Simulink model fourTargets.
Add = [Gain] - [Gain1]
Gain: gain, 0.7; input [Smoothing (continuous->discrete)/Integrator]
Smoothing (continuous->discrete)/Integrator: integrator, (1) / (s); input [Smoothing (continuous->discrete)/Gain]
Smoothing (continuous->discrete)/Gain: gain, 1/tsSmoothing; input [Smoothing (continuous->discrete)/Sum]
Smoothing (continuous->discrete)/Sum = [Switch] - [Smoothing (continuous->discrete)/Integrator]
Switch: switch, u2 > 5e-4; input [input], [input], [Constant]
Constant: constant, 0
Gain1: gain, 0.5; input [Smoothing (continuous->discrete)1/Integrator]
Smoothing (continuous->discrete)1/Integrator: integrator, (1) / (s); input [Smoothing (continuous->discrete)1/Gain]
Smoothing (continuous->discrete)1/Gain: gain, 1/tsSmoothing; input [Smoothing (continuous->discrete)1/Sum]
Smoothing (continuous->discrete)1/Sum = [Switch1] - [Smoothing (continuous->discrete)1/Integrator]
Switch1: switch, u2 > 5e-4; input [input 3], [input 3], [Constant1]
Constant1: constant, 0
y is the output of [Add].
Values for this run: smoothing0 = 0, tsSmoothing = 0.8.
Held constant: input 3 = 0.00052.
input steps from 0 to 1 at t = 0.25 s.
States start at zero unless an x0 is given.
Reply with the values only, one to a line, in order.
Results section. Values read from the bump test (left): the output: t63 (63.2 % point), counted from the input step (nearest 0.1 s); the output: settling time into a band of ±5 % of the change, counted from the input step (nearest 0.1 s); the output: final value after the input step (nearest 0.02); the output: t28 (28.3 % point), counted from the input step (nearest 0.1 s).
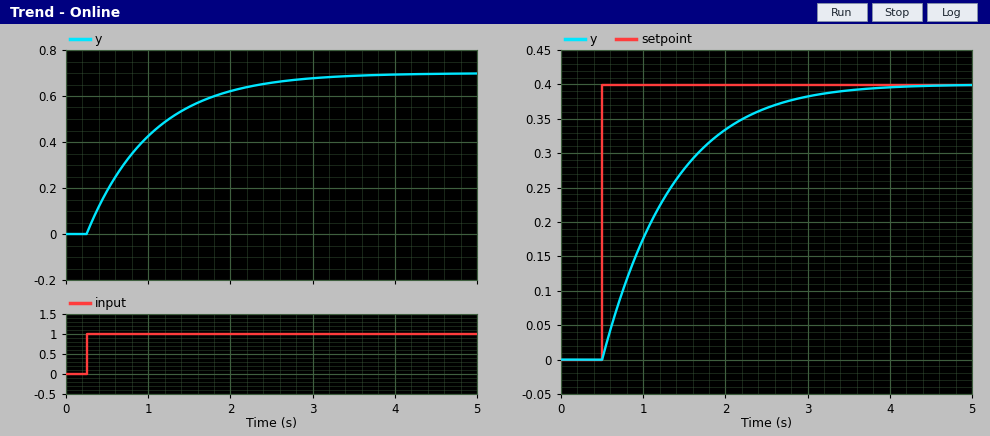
0.8 s
2.4 s
0.70
0.3 s
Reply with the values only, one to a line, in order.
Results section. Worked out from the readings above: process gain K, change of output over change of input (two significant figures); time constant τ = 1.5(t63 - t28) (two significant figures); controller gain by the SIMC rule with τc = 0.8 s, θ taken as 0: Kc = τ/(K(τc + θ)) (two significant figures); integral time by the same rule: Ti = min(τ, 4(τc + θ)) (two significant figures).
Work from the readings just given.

0.70
0.75 s
1.3
0.75 s
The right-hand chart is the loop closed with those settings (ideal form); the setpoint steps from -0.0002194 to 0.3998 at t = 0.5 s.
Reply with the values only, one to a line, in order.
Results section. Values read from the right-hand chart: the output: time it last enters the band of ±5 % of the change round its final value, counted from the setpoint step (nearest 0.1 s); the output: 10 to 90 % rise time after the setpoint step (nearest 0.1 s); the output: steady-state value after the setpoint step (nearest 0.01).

2.4 s
1.8 s
0.40
